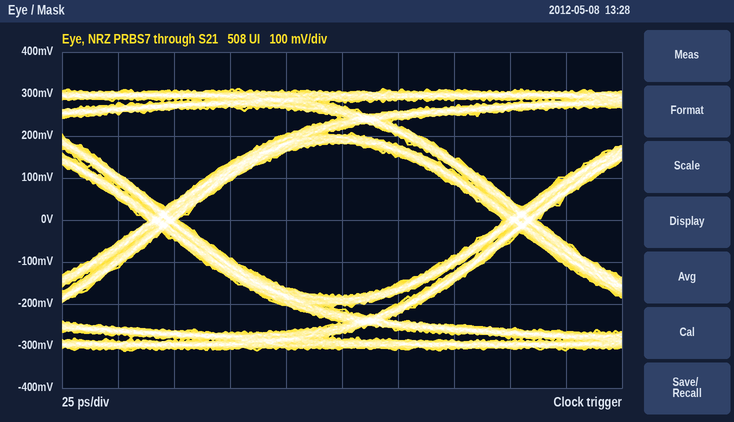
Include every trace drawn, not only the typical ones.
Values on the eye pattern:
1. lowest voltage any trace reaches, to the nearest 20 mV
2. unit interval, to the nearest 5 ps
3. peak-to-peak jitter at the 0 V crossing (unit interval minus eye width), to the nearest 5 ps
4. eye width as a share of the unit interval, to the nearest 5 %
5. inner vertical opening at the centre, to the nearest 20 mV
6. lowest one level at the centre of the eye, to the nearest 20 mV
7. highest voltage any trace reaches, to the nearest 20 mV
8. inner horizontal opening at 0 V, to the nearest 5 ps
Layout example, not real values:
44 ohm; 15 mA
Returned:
-320 mV; 160 ps; 15 ps; 90 %; 360 mV; 180 mV; 320 mV; 145 ps
